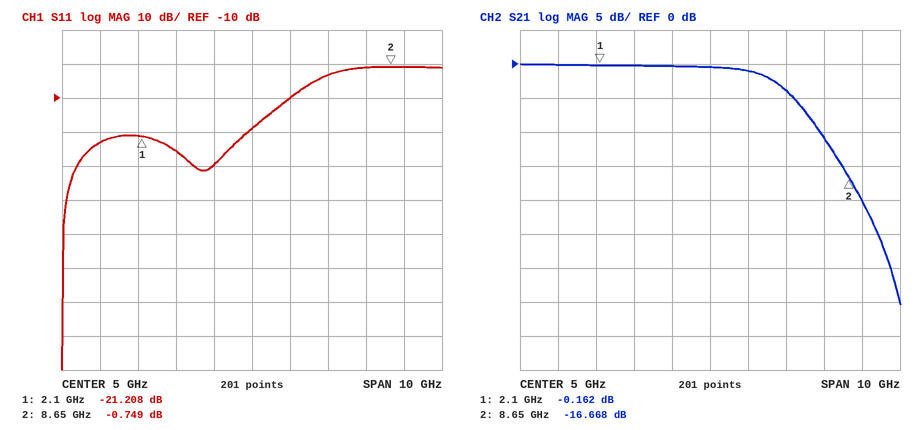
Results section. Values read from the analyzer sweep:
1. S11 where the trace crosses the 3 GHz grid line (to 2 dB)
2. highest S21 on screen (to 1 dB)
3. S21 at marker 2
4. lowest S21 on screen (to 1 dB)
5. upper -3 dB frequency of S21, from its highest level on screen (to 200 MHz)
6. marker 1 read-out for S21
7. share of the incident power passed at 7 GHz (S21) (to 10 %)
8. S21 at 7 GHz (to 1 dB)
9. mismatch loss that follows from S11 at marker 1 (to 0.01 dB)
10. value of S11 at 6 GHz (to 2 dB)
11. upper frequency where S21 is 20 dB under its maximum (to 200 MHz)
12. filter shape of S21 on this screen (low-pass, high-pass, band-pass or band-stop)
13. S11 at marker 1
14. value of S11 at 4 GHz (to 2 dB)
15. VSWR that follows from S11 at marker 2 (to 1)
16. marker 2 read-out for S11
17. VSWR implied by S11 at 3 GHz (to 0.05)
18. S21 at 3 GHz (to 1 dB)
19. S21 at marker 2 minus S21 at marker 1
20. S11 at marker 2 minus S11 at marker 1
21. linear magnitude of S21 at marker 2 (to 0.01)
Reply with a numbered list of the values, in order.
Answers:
1. -26 dB
2. 0 dB
3. -16.668 dB
4. -35 dB
5. 6.8 GHz
6. -0.162 dB
7. 40 %
8. -4 dB
9. 0.03 dB
10. -10 dB
11. 9.0 GHz
12. low-pass
13. -21.208 dB
14. -30 dB
15. 23
16. -0.749 dB
17. 1.10
18. 0 dB
19. -16.506 dB
20. 20.459 dB
21. 0.15
